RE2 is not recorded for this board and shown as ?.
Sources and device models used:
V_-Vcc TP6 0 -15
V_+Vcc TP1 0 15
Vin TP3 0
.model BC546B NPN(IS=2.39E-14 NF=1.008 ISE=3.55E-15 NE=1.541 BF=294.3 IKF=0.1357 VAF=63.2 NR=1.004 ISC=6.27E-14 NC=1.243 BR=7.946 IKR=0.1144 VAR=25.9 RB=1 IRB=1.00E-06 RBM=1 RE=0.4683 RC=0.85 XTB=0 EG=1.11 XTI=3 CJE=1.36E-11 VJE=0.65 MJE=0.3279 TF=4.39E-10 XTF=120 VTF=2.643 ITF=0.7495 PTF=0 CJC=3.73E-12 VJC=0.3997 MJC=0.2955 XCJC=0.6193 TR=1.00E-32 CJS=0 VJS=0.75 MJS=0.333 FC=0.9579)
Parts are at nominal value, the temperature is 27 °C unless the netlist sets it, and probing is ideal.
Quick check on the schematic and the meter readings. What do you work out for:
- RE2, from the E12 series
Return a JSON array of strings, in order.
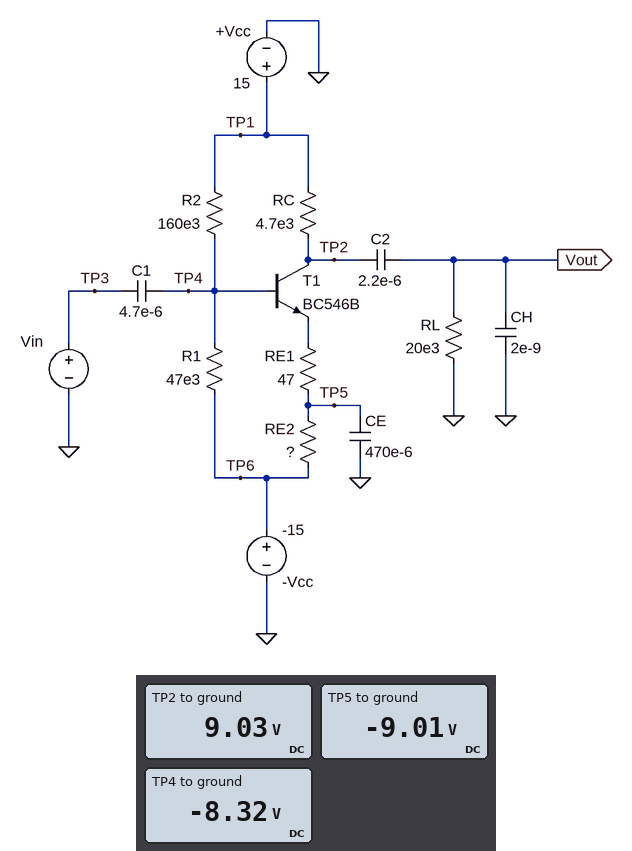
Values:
["4.7 kΩ"]
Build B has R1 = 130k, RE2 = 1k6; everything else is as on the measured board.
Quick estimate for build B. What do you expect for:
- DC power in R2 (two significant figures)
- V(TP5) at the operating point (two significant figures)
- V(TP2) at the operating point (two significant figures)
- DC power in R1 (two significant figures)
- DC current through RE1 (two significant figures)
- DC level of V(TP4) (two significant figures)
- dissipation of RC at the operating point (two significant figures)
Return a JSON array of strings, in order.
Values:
["2.9 mW", "-7.4 V", "-7.1 V", "560 µW", "4.8 mA", "-6.5 V", "100 mW"]
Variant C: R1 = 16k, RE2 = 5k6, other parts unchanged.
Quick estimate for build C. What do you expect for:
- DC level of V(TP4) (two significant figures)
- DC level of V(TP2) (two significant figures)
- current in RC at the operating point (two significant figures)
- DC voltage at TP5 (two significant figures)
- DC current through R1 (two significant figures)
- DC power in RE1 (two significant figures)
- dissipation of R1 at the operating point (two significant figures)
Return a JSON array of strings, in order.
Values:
["-12 V", "13 V", "370 µA", "-13 V", "170 µA", "6.6 µW", "460 µW"]
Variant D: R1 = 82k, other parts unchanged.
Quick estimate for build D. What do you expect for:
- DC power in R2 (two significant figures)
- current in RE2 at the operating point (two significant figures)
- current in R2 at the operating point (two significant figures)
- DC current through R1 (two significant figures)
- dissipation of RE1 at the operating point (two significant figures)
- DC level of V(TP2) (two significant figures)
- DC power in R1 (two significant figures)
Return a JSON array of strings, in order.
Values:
["2.5 mW", "1.9 mA", "130 µA", "120 µA", "180 µW", "5.9 V", "1.2 mW"]
